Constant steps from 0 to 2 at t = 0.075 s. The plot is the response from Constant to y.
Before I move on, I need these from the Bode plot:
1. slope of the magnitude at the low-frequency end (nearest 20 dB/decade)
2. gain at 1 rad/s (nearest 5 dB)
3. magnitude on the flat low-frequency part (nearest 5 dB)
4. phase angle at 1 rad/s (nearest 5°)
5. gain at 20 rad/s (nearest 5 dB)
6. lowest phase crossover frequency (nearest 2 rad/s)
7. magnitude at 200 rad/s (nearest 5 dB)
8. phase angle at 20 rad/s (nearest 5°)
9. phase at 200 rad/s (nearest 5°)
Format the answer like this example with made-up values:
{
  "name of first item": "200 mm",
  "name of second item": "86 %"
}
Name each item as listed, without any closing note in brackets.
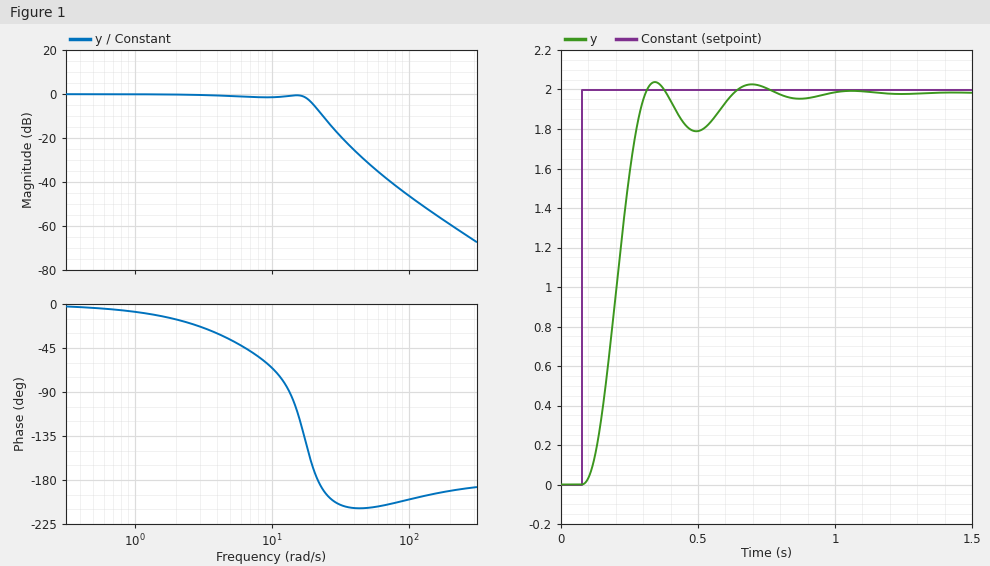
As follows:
{
  "slope of the magnitude at the low-frequency end": "0 dB/decade",
  "gain at 1 rad/s": "0 dB",
  "magnitude on the flat low-frequency part": "0 dB",
  "phase angle at 1 rad/s": "-10°",
  "gain at 20 rad/s": "-5 dB",
  "lowest phase crossover frequency": "22 rad/s",
  "magnitude at 200 rad/s": "-60 dB",
  "phase angle at 20 rad/s": "-165°",
  "phase at 200 rad/s": "-190°"
}
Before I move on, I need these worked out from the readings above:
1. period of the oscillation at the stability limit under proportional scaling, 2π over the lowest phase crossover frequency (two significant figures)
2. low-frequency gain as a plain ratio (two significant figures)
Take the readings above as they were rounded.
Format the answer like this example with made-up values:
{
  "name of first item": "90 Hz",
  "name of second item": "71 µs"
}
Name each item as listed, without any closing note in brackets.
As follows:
{
  "period of the oscillation at the stability limit under proportional scaling, 2π over the lowest phase crossover frequency": "0.29 s",
  "low-frequency gain as a plain ratio": "1.0"
}
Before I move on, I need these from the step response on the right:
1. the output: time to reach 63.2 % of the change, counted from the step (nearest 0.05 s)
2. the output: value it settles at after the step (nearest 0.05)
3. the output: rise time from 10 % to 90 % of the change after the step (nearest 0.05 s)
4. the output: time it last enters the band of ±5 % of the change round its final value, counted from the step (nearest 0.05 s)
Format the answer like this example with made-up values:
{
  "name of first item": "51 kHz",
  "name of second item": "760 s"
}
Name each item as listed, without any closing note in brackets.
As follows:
{
  "the output: time to reach 63.2 % of the change, counted from the step": "0.15 s",
  "the output: value it settles at after the step": "2.00",
  "the output: rise time from 10 % to 90 % of the change after the step": "0.15 s",
  "the output: time it last enters the band of ±5 % of the change round its final value, counted from the step": "0.50 s"
}
